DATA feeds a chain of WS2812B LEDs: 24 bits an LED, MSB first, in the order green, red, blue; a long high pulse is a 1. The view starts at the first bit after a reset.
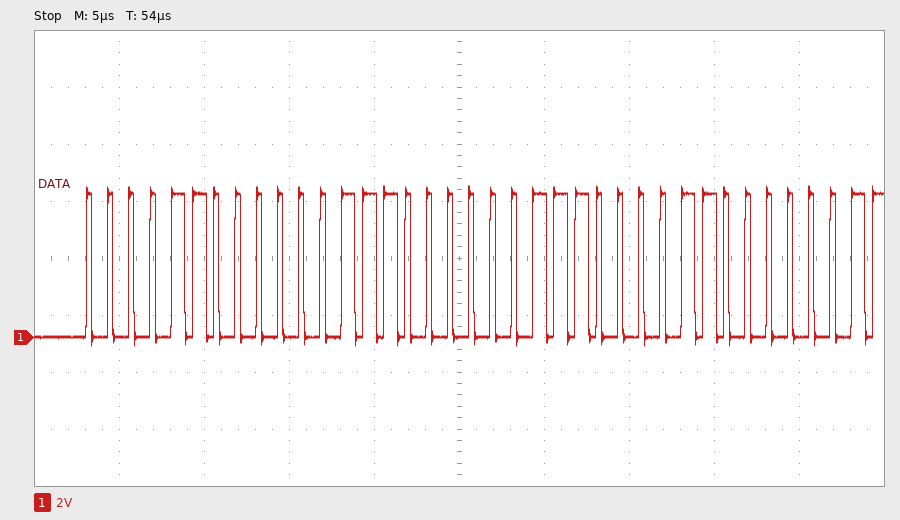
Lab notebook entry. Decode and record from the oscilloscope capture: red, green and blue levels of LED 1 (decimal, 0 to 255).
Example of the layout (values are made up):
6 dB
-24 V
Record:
14, 12, 7
